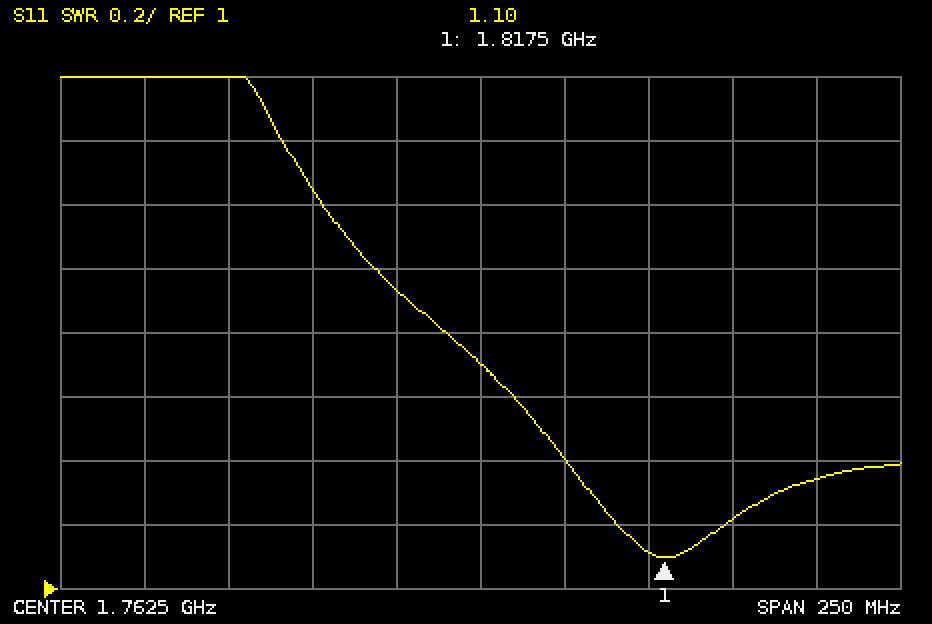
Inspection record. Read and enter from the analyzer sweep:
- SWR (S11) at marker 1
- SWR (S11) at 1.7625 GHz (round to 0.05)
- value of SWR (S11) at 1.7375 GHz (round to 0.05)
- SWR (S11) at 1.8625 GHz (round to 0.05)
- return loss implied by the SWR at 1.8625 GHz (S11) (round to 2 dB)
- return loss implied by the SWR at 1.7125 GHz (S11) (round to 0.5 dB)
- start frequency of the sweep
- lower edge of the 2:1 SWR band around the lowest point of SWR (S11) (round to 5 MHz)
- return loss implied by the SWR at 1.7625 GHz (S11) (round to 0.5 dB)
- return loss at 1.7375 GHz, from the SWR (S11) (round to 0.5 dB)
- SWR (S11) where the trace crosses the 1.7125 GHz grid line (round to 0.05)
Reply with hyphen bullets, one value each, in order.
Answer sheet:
- 1.10
- 1.70
- 1.95
- 1.35
- 16 dB
- 8.5 dB
- 1.6375 GHz
- 1.730 GHz
- 11.5 dB
- 10.0 dB
- 2.25
